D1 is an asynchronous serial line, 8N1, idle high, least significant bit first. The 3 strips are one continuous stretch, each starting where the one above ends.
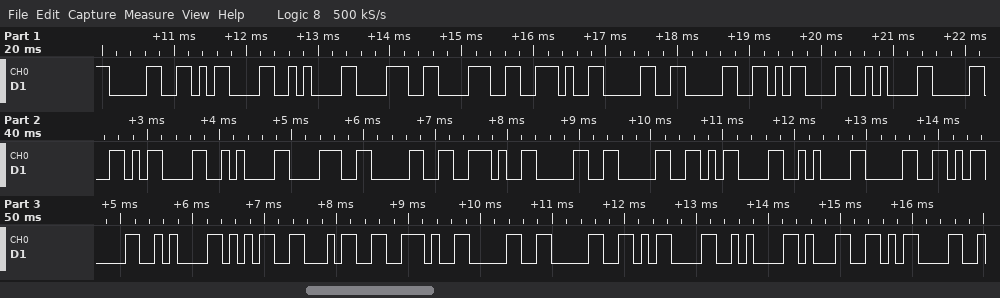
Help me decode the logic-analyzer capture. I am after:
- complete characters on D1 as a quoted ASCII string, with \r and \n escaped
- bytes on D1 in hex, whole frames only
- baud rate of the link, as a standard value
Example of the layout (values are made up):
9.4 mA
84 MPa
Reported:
"0\r\n88.00\r\n0\r\n80.00\r\n0\r\n54.00\r\n1\r"
30 0D 0A 38 38 2E 30 30 0D 0A 30 0D 0A 38 30 2E 30 30 0D 0A 30 0D 0A 35 34 2E 30 30 0D 0A 31 0D
9600 baud
